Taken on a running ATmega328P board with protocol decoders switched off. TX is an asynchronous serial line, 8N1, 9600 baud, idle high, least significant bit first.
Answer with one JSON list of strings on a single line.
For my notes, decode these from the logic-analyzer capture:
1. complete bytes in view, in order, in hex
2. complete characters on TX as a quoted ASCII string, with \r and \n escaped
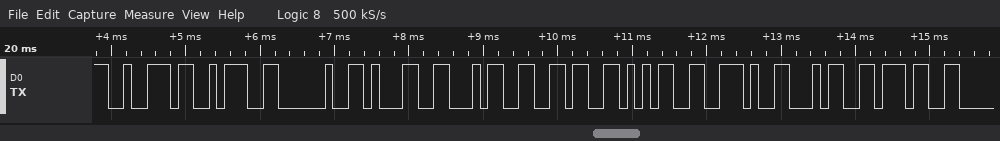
["0x72 0x3A 0x20 0x31 0x34 0x36 0x35 0x2E 0x34 0x37", "\"r: 1465.47\""]
